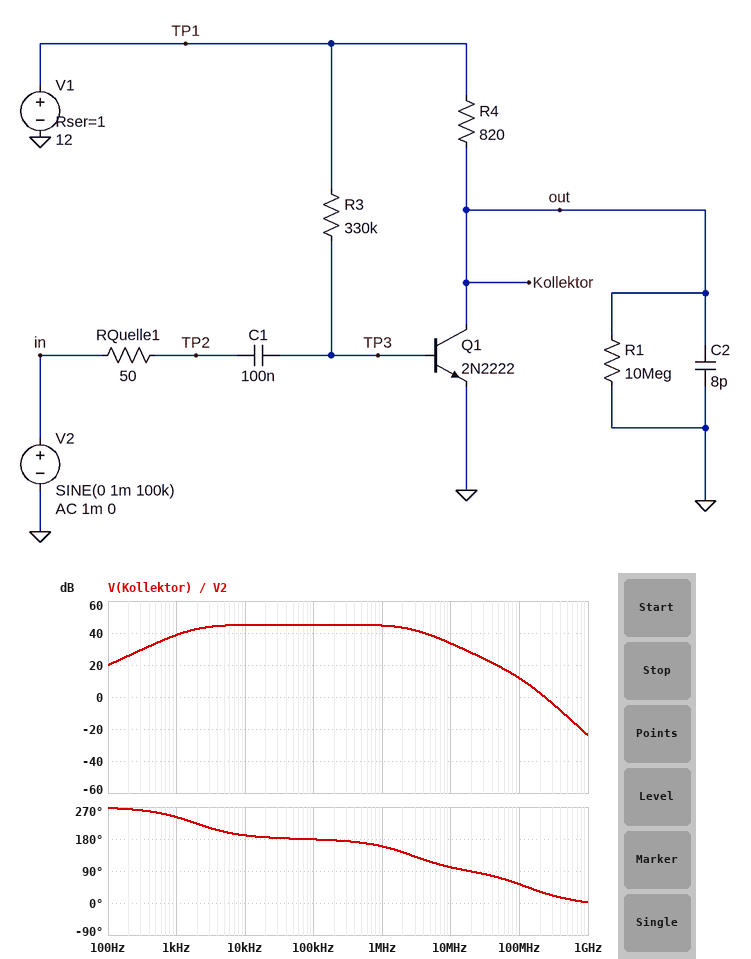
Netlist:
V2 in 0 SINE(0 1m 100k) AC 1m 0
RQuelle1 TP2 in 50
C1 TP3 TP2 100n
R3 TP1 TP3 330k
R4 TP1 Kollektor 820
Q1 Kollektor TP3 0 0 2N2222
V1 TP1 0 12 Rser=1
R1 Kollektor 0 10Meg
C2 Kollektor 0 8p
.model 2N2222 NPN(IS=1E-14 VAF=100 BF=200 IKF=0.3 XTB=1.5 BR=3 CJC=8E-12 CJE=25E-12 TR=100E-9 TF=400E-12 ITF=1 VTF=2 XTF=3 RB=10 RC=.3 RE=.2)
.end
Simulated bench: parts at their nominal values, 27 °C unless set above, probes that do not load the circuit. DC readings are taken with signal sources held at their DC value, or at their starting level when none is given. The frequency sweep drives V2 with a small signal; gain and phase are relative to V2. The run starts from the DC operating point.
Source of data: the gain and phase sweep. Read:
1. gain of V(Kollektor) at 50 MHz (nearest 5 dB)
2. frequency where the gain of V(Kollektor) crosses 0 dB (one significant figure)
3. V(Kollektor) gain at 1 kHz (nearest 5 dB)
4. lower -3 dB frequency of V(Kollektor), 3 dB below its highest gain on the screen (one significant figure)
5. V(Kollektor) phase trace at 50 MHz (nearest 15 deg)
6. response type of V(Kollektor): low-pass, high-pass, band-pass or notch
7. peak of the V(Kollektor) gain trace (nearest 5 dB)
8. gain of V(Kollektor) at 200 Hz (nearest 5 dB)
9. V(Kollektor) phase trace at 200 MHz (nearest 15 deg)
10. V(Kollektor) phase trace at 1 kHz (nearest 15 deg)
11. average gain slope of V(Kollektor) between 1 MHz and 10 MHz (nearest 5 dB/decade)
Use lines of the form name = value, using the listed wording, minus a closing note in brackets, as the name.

gain of V(Kollektor) at 50 MHz = 20 dB
frequency where the gain of V(Kollektor) crosses 0 dB = 200 MHz
V(Kollektor) gain at 1 kHz = 40 dB
lower -3 dB frequency of V(Kollektor), 3 dB below its highest gain on the screen = 2 kHz
V(Kollektor) phase trace at 50 MHz = 75 deg
response type of V(Kollektor): low-pass, high-pass, band-pass or notch = band-pass
peak of the V(Kollektor) gain trace = 45 dB
gain of V(Kollektor) at 200 Hz = 25 dB
V(Kollektor) phase trace at 200 MHz = 30 deg
V(Kollektor) phase trace at 1 kHz = 240 deg
average gain slope of V(Kollektor) between 1 MHz and 10 MHz = -10 dB/decade
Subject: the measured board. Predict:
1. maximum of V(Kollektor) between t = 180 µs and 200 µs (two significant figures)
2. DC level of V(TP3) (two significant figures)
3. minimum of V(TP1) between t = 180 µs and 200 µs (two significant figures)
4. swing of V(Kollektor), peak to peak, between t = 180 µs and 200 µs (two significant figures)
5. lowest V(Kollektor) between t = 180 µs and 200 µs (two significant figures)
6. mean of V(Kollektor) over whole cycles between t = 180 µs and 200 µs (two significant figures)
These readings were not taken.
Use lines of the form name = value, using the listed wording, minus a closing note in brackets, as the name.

maximum of V(Kollektor) between t = 180 µs and 200 µs = 6.4 V
DC level of V(TP3) = 710 mV
minimum of V(TP1) between t = 180 µs and 200 µs = 12 V
swing of V(Kollektor), peak to peak, between t = 180 µs and 200 µs = 360 mV
lowest V(Kollektor) between t = 180 µs and 200 µs = 6.0 V
mean of V(Kollektor) over whole cycles between t = 180 µs and 200 µs = 6.2 V
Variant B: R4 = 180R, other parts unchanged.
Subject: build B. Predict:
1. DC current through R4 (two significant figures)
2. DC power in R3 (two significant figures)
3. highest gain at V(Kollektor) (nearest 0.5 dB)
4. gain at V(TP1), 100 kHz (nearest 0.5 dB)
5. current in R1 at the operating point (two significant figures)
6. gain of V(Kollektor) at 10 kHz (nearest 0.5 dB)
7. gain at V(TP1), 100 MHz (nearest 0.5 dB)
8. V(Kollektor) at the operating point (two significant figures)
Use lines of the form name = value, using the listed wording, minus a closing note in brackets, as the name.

DC current through R4 = 7.4 mA
DC power in R3 = 390 µW
highest gain at V(Kollektor) = 33.0 dB
gain at V(TP1), 100 kHz = -12.5 dB
current in R1 at the operating point = 1.1 µA
gain of V(Kollektor) at 10 kHz = 32.5 dB
gain at V(TP1), 100 MHz = -34.5 dB
V(Kollektor) at the operating point = 11 V
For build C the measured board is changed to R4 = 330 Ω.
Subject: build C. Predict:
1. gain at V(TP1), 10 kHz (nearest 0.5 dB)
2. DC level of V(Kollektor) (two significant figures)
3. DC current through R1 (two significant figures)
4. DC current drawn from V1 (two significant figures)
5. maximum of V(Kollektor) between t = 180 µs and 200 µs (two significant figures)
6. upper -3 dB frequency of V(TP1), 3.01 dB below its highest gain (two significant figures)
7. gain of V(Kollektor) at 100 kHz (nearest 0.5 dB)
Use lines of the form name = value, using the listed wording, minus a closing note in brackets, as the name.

gain at V(TP1), 10 kHz = -12.5 dB
DC level of V(Kollektor) = 9.6 V
DC current through R1 = 960 nA
DC current drawn from V1 = 7.3 mA
maximum of V(Kollektor) between t = 180 µs and 200 µs = 9.7 V
upper -3 dB frequency of V(TP1), 3.01 dB below its highest gain = 5.9 MHz
gain of V(Kollektor) at 100 kHz = 38.0 dB
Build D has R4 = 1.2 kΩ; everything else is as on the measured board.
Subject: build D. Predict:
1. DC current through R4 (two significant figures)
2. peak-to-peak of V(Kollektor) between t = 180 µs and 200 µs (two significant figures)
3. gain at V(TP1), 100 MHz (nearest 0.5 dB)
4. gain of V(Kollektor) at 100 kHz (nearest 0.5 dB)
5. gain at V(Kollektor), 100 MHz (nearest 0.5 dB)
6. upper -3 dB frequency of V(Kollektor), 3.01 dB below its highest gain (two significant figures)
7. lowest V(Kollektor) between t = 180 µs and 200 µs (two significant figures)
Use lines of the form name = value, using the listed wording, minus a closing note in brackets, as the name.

DC current through R4 = 6.9 mA
peak-to-peak of V(Kollektor) between t = 180 µs and 200 µs = 510 mV
gain at V(TP1), 100 MHz = -50.5 dB
gain of V(Kollektor) at 100 kHz = 48.0 dB
gain at V(Kollektor), 100 MHz = 11.0 dB
upper -3 dB frequency of V(Kollektor), 3.01 dB below its highest gain = 1.7 MHz
lowest V(Kollektor) between t = 180 µs and 200 µs = 3.5 V
